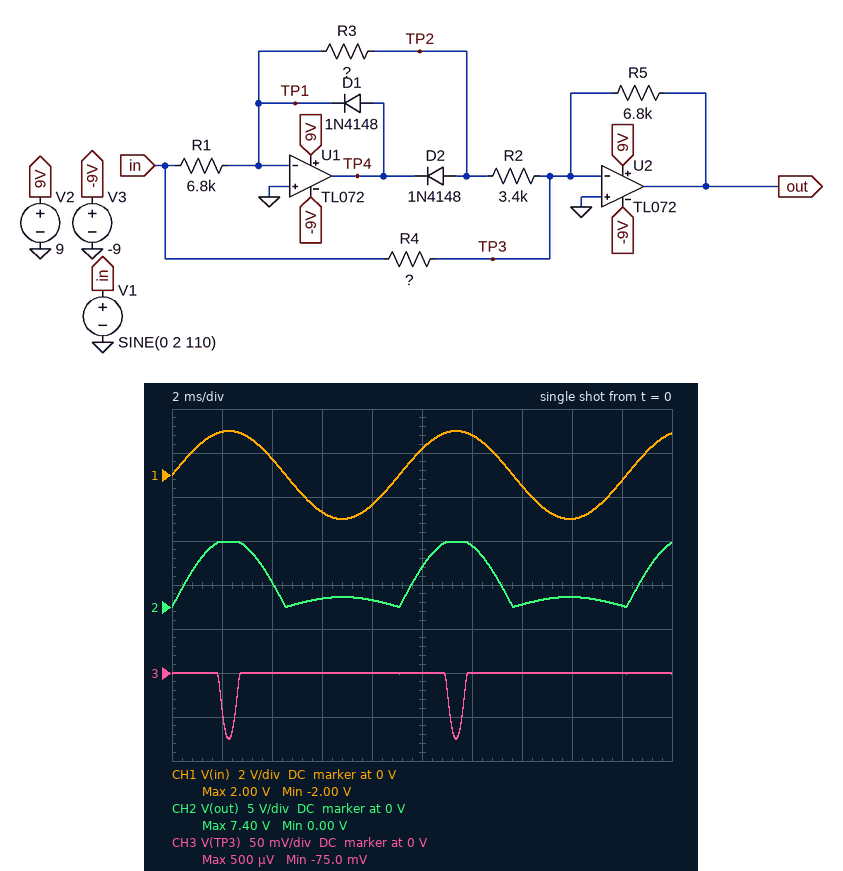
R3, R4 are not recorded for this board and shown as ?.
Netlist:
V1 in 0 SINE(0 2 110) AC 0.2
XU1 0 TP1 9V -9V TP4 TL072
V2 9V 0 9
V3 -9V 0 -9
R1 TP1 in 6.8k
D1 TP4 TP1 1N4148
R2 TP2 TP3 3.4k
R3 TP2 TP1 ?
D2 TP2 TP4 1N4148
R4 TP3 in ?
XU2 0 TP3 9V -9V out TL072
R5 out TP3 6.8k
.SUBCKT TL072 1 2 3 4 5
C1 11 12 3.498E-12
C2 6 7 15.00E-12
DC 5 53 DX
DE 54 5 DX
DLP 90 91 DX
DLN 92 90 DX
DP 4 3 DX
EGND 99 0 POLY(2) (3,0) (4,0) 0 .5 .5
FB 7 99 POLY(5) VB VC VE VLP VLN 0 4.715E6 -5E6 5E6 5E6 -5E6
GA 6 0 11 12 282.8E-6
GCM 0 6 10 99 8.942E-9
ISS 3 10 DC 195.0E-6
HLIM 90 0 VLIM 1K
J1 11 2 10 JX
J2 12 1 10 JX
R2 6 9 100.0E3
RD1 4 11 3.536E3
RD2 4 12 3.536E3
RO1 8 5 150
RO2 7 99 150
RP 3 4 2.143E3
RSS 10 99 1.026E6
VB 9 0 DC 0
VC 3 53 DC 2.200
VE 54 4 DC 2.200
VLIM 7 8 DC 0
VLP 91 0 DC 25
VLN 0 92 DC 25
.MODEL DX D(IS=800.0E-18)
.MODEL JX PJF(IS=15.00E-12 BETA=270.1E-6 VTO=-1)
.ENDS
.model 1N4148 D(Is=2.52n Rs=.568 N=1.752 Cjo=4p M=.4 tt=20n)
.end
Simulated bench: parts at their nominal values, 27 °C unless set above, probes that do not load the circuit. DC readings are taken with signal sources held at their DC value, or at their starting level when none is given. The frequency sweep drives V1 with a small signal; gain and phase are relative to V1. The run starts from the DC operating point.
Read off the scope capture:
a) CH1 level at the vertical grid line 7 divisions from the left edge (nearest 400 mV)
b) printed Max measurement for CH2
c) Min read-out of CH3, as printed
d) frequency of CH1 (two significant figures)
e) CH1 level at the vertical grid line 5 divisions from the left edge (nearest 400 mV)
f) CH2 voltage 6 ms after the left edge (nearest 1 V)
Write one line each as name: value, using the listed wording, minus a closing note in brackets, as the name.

CH1 level at the vertical grid line 7 divisions from the left edge: -400 mV
printed Max measurement for CH2: 7.40 V
Min read-out of CH3, as printed: -75.0 mV
frequency of CH1: 110 Hz
CH1 level at the vertical grid line 5 divisions from the left edge: 1.2 V
CH2 voltage 6 ms after the left edge: 1 V
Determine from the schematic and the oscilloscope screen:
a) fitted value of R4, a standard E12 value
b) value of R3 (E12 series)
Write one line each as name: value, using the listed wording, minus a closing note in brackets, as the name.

fitted value of R4, a standard E12 value: 12 kΩ
value of R3: 15 kΩ
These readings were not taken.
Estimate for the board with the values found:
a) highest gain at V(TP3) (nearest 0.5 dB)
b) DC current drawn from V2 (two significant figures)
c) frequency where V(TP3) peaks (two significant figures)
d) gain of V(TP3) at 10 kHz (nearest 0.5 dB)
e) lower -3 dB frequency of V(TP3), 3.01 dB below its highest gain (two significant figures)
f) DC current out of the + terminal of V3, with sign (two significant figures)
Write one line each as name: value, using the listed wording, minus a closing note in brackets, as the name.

highest gain at V(TP3): -8.0 dB
DC current drawn from V2: 17 mA
frequency where V(TP3) peaks: 4.5 MHz
gain of V(TP3) at 10 kHz: -56.5 dB
lower -3 dB frequency of V(TP3), 3.01 dB below its highest gain: 2.0 MHz
DC current out of the + terminal of V3, with sign: -17 mA
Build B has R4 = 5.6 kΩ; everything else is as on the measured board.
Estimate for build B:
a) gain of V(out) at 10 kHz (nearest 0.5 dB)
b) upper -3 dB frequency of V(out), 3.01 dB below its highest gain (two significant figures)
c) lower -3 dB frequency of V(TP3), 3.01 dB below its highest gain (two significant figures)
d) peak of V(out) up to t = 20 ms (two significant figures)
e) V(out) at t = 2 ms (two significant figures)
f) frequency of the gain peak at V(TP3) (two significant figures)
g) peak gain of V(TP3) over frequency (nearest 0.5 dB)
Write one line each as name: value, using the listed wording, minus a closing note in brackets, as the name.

gain of V(out) at 10 kHz: 1.5 dB
upper -3 dB frequency of V(out), 3.01 dB below its highest gain: 1.8 MHz
lower -3 dB frequency of V(TP3), 3.01 dB below its highest gain: 1.4 MHz
peak of V(out) up to t = 20 ms: 6.4 V
V(out) at t = 2 ms: 6.3 V
frequency of the gain peak at V(TP3): 4.1 MHz
peak gain of V(TP3) over frequency: -5.0 dB
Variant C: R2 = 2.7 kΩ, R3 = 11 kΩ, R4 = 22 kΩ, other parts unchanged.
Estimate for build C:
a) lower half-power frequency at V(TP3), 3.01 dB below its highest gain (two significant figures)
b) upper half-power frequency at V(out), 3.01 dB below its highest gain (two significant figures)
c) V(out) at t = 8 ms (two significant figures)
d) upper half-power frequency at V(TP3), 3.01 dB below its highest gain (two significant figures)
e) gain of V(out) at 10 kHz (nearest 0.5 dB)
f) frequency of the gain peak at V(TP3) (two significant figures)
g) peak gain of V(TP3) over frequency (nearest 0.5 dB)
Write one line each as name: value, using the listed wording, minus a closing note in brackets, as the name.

lower half-power frequency at V(TP3), 3.01 dB below its highest gain: 2.2 MHz
upper half-power frequency at V(out), 3.01 dB below its highest gain: 3.7 MHz
V(out) at t = 8 ms: 420 mV
upper half-power frequency at V(TP3), 3.01 dB below its highest gain: 9.6 MHz
gain of V(out) at 10 kHz: -10.0 dB
frequency of the gain peak at V(TP3): 4.7 MHz
peak gain of V(TP3) over frequency: -10.5 dB
